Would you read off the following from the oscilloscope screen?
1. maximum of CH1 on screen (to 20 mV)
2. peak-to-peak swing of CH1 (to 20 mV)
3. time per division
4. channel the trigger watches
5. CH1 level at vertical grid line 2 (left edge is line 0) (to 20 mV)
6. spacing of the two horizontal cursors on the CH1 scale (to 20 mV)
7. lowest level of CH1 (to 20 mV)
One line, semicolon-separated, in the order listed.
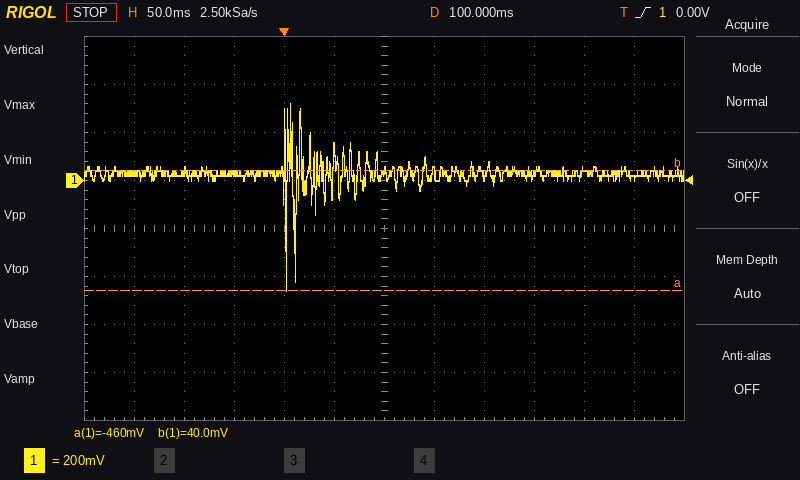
320 mV; 780 mV; 50 ms; CH1; 40 mV; 500 mV; -460 mV
